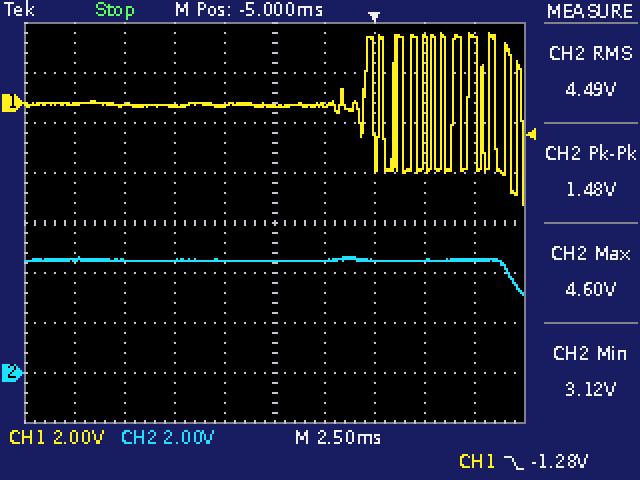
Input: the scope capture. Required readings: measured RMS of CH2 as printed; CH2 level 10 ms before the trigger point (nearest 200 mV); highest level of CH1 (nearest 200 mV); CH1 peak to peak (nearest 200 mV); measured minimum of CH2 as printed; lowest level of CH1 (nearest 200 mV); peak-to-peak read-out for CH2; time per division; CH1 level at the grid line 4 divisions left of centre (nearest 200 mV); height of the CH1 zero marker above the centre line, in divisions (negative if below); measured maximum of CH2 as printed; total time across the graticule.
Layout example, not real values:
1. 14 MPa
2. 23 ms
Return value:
1. 4.49 V
2. 4.6 V
3. 2.8 V
4. 6.8 V
5. 3.12 V
6. -4.0 V
7. 1.48 V
8. 2.5 ms
9. 0.0 V
10. +2.4 div
11. 4.60 V
12. 25 ms
